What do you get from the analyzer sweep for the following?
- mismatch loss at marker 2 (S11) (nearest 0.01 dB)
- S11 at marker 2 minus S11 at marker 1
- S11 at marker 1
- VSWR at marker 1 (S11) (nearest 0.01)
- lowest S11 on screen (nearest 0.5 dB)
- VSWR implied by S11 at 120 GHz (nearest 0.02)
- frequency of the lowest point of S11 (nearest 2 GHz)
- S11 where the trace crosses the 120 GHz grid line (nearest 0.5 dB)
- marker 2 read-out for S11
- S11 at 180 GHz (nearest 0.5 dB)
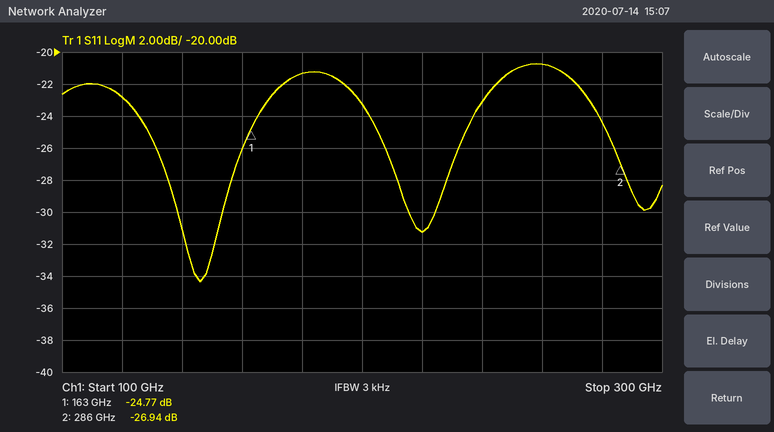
0.01 dB
-2.17 dB
-24.77 dB
1.12
-34.5 dB
1.16
146 GHz
-23.0 dB
-26.94 dB
-21.5 dB
